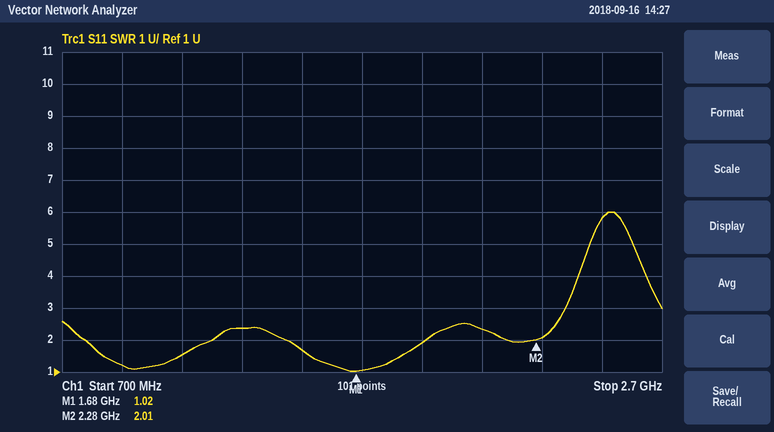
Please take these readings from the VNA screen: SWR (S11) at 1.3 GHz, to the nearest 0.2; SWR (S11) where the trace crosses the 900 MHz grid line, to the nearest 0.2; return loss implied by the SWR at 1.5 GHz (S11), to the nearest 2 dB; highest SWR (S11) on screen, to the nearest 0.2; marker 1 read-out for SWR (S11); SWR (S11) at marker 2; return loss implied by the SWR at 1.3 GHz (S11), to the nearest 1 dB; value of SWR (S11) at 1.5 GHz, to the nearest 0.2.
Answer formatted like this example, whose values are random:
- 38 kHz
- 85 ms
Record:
- 2.4
- 1.2
- 12 dB
- 6.0
- 1.02
- 2.01
- 8 dB
- 1.6
